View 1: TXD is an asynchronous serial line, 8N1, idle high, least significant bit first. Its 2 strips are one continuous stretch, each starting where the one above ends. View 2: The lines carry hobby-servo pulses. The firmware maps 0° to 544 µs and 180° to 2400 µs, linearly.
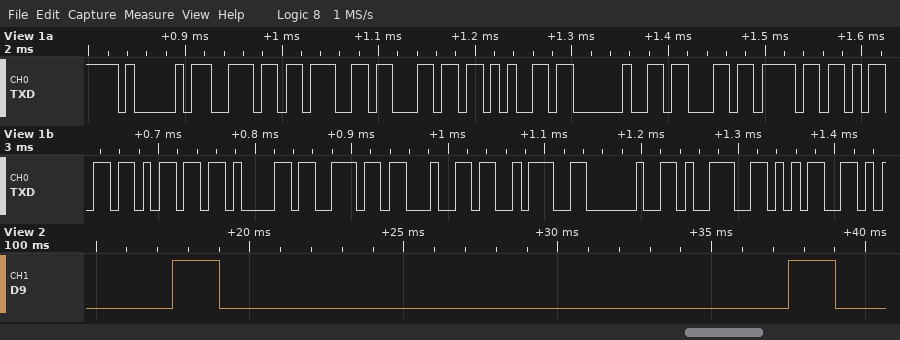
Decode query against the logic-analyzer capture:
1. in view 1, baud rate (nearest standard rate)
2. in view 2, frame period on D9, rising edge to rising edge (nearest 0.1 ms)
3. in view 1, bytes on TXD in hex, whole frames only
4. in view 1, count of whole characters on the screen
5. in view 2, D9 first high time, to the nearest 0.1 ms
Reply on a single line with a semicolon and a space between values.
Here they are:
115200 baud; 20.0 ms; 41 6E 67 6C 65 20 63 6F 6D 6D 61 6E 64 3A 20 39 35; 17; 1.5 ms
